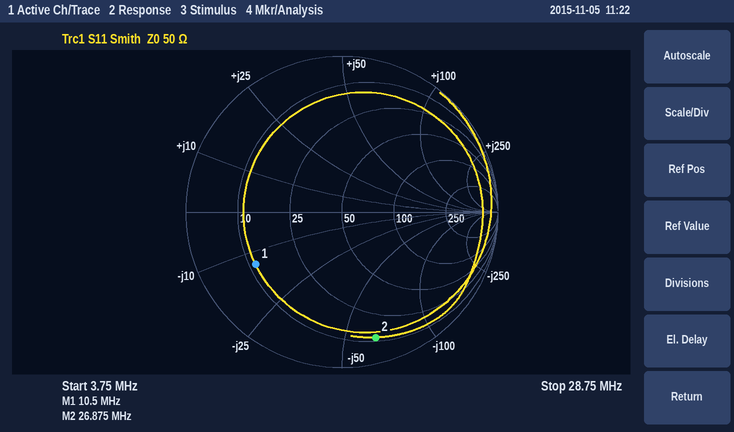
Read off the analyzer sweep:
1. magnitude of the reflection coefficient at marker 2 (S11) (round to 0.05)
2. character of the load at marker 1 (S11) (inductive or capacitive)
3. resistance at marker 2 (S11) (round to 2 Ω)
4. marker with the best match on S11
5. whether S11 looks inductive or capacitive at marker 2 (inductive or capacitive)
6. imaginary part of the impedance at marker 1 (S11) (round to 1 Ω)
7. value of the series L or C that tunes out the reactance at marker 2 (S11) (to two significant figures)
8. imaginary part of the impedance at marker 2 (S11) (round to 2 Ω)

0.85
capacitive
12 Ω
marker 1
capacitive
-13 Ω
380 nH
-64 Ω
